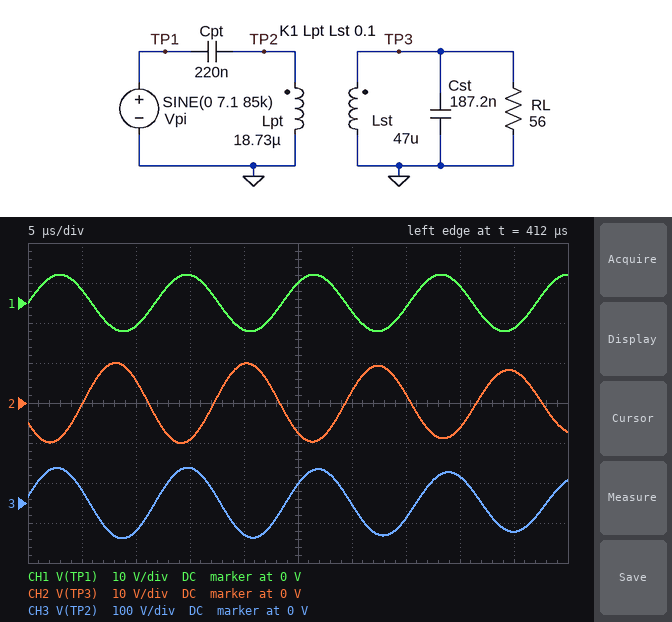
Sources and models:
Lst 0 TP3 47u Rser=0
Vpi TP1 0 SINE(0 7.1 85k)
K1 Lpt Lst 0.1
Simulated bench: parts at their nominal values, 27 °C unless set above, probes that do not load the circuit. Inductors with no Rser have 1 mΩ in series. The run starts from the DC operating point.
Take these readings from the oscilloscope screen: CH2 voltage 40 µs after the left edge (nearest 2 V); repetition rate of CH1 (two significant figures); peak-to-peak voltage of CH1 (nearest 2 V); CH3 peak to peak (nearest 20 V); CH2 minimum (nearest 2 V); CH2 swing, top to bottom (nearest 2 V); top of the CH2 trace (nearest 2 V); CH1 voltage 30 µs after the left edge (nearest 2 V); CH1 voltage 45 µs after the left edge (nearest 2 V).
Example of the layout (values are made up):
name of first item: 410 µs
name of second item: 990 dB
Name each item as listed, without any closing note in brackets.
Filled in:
CH2 voltage 40 µs after the left edge: -6 V
repetition rate of CH1: 85 kHz
peak-to-peak voltage of CH1: 14 V
CH3 peak to peak: 180 V
CH2 minimum: -10 V
CH2 swing, top to bottom: 20 V
top of the CH2 trace: 10 V
CH1 voltage 30 µs after the left edge: -2 V
CH1 voltage 45 µs after the left edge: -6 V
